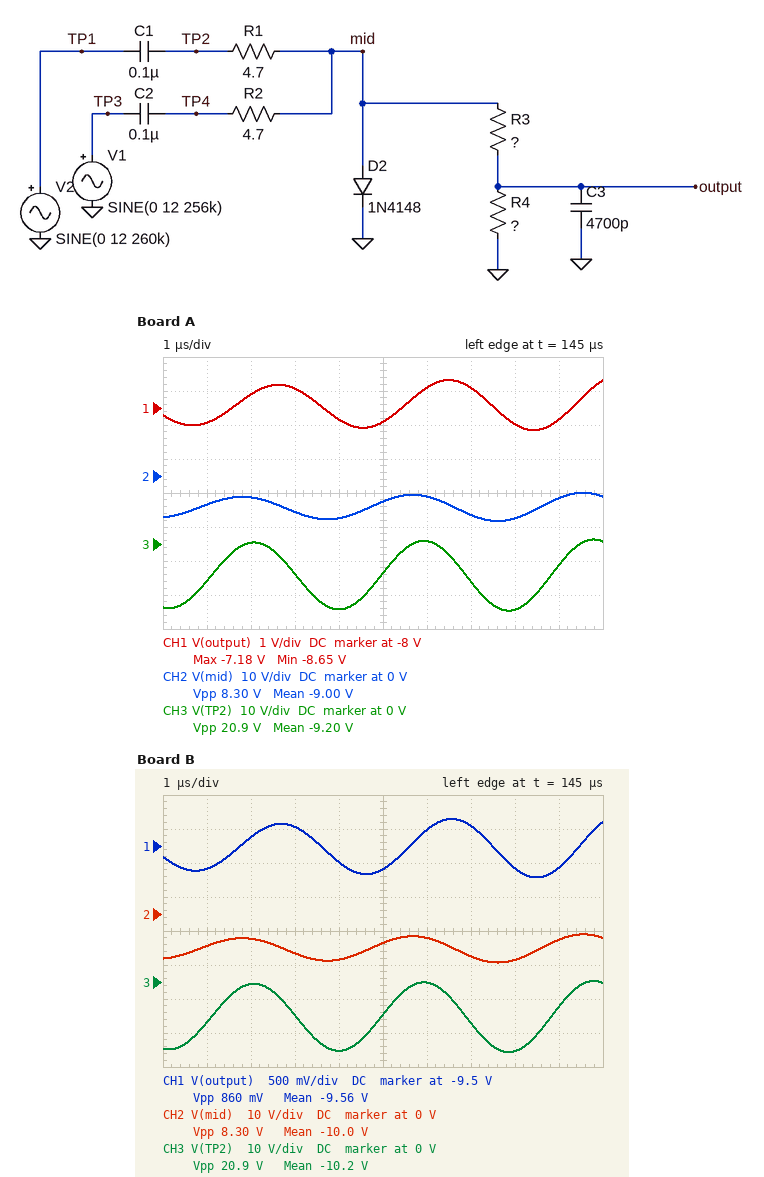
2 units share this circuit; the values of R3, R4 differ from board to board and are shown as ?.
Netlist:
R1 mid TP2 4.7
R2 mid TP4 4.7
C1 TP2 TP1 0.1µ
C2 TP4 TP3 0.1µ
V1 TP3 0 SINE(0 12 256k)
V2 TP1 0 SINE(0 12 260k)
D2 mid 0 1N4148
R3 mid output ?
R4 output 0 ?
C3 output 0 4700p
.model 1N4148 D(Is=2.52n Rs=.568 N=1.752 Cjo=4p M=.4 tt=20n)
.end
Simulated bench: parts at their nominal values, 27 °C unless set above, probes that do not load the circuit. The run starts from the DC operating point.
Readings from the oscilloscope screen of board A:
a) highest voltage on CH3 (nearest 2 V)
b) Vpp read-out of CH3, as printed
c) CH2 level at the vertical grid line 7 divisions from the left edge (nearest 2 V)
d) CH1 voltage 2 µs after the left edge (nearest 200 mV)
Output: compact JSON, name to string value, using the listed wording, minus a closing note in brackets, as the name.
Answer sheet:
{"highest voltage on CH3": "2 V", "Vpp read-out of CH3, as printed": "20.9 V", "CH2 level at the vertical grid line 7 divisions from the left edge": "-12 V", "CH1 voltage 2 µs after the left edge": "-7.6 V"}
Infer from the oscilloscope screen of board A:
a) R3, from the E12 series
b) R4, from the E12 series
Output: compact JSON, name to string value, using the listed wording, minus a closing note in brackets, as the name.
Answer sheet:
{"R3, from the E12 series": "680 Ω", "R4, from the E12 series": "3.9 kΩ"}
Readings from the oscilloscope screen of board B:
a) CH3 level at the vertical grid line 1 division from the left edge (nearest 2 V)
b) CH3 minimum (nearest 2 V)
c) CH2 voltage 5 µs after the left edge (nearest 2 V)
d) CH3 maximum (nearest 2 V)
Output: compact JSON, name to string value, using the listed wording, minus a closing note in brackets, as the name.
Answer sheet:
{"CH3 level at the vertical grid line 1 division from the left edge": "-12 V", "CH3 minimum": "-20 V", "CH2 voltage 5 µs after the left edge": "-8 V", "CH3 maximum": "0 V"}
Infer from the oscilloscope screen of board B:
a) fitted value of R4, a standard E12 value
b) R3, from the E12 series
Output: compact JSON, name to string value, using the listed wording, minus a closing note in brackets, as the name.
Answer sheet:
{"fitted value of R4, a standard E12 value": "15 kΩ", "R3, from the E12 series": "1.2 kΩ"}
